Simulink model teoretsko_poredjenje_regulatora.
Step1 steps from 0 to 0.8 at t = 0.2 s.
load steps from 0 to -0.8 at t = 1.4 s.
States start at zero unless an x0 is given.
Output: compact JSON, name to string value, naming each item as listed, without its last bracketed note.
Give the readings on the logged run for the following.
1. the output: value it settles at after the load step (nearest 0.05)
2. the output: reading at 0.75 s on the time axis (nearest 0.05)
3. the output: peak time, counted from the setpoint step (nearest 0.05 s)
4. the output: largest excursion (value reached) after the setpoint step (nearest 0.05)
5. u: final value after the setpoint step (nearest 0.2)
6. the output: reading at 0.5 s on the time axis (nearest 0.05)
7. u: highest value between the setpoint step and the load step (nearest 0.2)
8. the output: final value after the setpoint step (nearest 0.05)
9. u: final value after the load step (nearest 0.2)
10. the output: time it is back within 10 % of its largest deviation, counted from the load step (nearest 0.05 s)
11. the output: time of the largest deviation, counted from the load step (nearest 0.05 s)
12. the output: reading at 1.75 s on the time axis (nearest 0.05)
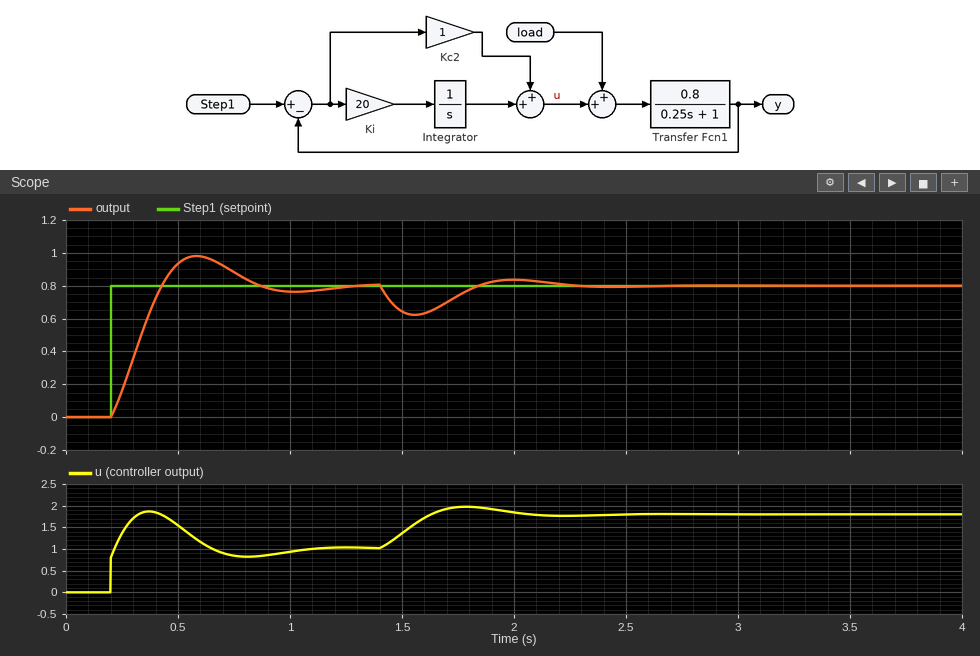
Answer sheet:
{"the output: value it settles at after the load step": "0.80", "the output: reading at 0.75 s on the time axis": "0.90", "the output: peak time, counted from the setpoint step": "0.40 s", "the output: largest excursion (value reached) after the setpoint step": "1.00", "u: final value after the setpoint step": "1.0", "the output: reading at 0.5 s on the time axis": "0.95", "u: highest value between the setpoint step and the load step": "1.8", "the output: final value after the setpoint step": "0.80", "u: final value after the load step": "1.8", "the output: time it is back within 10 % of its largest deviation, counted from the load step": "0.75 s", "the output: time of the largest deviation, counted from the load step": "0.15 s", "the output: reading at 1.75 s on the time axis": "0.75"}
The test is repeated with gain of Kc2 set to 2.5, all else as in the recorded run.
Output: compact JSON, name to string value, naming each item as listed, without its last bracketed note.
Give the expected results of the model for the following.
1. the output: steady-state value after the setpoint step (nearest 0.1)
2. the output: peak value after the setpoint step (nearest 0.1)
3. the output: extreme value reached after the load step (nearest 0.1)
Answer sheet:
{"the output: steady-state value after the setpoint step": "0.8", "the output: peak value after the setpoint step": "0.9", "the output: extreme value reached after the load step": "0.7"}
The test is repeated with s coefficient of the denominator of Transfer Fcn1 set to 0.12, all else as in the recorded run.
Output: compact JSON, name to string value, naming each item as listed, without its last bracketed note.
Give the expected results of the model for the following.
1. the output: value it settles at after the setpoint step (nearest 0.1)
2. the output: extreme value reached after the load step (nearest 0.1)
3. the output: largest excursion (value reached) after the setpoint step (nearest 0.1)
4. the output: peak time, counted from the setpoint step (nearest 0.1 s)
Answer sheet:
{"the output: value it settles at after the setpoint step": "0.8", "the output: extreme value reached after the load step": "0.6", "the output: largest excursion (value reached) after the setpoint step": "0.9", "the output: peak time, counted from the setpoint step": "0.3 s"}
